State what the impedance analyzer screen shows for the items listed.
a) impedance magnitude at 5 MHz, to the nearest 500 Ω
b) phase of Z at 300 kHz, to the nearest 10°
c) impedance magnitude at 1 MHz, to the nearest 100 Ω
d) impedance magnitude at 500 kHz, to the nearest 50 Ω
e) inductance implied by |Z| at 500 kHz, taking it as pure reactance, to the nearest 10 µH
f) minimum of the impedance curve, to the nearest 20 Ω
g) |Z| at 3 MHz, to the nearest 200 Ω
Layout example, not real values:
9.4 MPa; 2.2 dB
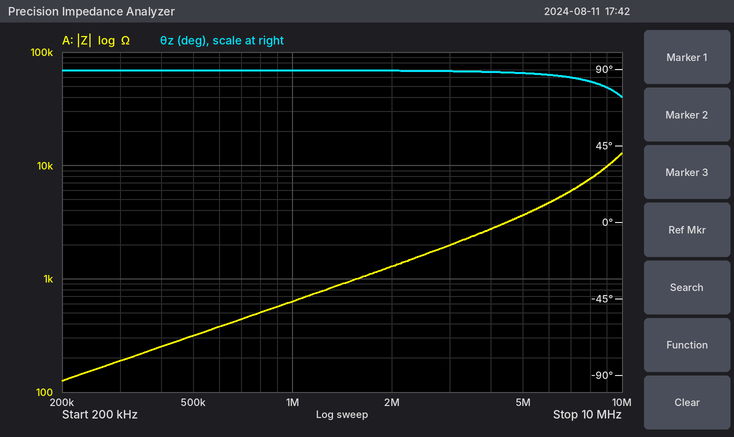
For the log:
3.5 kΩ; 90°; 600 Ω; 300 Ω; 100 µH; 120 Ω; 2.0 kΩ
